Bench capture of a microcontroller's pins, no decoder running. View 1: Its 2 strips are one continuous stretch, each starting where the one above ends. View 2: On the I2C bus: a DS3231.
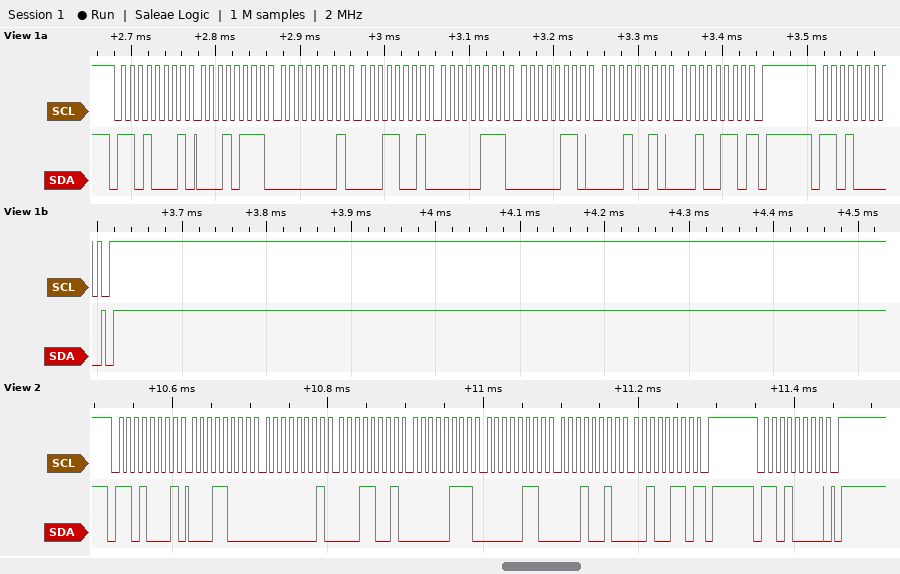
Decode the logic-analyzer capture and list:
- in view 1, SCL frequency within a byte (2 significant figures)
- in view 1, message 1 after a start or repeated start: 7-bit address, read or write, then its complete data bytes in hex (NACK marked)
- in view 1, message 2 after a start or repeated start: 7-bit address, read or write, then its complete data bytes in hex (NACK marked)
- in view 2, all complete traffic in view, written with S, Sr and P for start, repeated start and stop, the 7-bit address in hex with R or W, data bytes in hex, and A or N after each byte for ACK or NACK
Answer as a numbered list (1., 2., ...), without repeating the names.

1. 100 kHz
2. 0x68 read: 17 01 19 07 06 12 26 NACK
3. 0x68 write
4. S 68R A 18 A 01 A 19 A 07 A 06 A 12 A 26 N P S 68W A P
